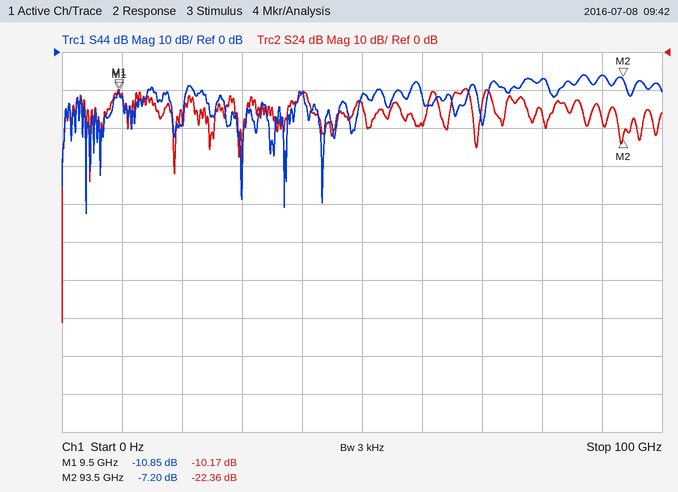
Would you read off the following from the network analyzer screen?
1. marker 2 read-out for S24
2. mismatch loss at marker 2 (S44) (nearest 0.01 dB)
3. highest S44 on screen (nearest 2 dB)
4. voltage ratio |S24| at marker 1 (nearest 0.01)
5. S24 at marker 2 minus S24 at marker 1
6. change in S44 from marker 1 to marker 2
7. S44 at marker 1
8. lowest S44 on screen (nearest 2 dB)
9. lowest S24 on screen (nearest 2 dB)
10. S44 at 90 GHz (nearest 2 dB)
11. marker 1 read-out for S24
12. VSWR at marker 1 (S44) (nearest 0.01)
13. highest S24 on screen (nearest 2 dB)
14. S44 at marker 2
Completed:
-22.36 dB
0.92 dB
-6 dB
0.31
-12.19 dB
3.65 dB
-10.85 dB
-42 dB
-72 dB
-6 dB
-10.17 dB
1.80
-10 dB
-7.20 dB
